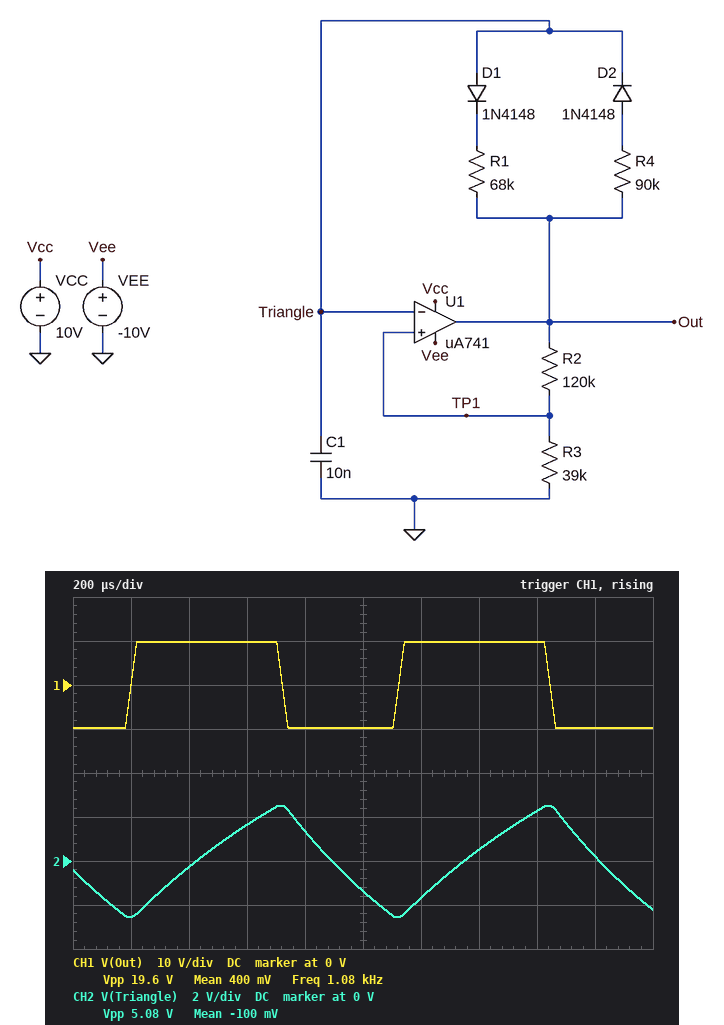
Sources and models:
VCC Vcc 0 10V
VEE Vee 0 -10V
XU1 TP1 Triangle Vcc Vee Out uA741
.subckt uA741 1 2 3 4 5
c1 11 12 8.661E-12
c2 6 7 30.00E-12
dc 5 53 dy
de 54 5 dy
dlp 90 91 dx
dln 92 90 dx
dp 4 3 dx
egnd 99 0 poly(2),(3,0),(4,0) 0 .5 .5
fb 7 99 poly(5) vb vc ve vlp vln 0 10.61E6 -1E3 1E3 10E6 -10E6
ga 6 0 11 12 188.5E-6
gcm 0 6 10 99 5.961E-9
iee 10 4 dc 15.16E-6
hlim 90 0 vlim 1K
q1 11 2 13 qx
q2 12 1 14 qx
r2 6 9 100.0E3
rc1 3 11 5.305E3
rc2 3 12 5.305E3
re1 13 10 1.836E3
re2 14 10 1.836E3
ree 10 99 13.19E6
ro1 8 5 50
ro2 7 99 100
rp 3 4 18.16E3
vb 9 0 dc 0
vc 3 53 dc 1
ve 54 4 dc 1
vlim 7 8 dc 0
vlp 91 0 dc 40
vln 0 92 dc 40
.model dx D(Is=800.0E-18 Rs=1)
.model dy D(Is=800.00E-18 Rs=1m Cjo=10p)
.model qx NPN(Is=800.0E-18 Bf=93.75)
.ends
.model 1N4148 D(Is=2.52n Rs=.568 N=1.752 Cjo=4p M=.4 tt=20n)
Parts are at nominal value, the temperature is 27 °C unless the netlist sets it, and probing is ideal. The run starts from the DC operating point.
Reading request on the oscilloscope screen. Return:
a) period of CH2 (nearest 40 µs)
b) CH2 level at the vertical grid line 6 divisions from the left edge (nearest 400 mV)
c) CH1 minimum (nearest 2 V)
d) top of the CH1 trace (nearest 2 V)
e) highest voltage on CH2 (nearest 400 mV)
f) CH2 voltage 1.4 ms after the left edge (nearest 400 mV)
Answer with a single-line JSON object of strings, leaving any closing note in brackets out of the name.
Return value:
{"period of CH2": "920 µs", "CH2 level at the vertical grid line 6 divisions from the left edge": "-1.6 V", "CH1 minimum": "-10 V", "top of the CH1 trace": "10 V", "highest voltage on CH2": "2.4 V", "CH2 voltage 1.4 ms after the left edge": "400 mV"}
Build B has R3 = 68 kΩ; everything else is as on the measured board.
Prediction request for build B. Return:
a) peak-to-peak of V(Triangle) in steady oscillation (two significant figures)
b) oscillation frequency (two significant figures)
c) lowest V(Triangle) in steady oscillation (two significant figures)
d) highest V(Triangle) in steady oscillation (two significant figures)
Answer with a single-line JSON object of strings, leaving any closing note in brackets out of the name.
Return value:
{"peak-to-peak of V(Triangle) in steady oscillation": "7.3 V", "oscillation frequency": "740 Hz", "lowest V(Triangle) in steady oscillation": "-3.7 V", "highest V(Triangle) in steady oscillation": "3.6 V"}
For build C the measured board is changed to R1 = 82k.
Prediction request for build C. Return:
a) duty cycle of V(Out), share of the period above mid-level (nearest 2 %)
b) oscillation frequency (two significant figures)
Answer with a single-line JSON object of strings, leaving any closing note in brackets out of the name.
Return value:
{"duty cycle of V(Out), share of the period above mid-level": "52 %", "oscillation frequency": "1.0 kHz"}
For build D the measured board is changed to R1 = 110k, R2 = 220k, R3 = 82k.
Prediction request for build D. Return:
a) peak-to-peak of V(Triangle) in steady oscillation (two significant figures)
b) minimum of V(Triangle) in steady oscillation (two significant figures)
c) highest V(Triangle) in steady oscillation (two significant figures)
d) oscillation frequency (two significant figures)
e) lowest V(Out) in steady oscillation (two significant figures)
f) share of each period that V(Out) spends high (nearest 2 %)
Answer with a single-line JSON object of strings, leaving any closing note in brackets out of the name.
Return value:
{"peak-to-peak of V(Triangle) in steady oscillation": "5.5 V", "minimum of V(Triangle) in steady oscillation": "-2.8 V", "highest V(Triangle) in steady oscillation": "2.8 V", "oscillation frequency": "790 Hz", "lowest V(Out) in steady oscillation": "-9.8 V", "share of each period that V(Out) spends high": "46 %"}
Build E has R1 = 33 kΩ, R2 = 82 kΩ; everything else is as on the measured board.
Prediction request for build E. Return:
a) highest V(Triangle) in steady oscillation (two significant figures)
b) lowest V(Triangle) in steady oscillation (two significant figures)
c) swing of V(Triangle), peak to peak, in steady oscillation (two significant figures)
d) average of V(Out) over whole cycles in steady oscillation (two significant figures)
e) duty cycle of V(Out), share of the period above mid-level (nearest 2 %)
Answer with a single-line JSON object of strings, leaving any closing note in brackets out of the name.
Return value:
{"highest V(Triangle) in steady oscillation": "3.3 V", "lowest V(Triangle) in steady oscillation": "-3.4 V", "swing of V(Triangle), peak to peak, in steady oscillation": "6.7 V", "average of V(Out) over whole cycles in steady oscillation": "4.3 V", "duty cycle of V(Out), share of the period above mid-level": "72 %"}
